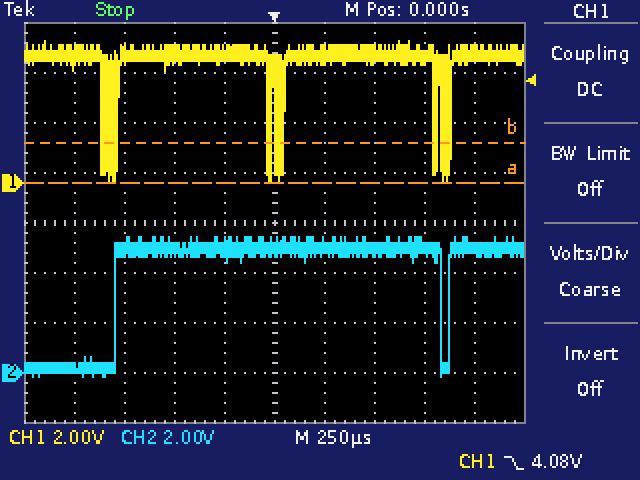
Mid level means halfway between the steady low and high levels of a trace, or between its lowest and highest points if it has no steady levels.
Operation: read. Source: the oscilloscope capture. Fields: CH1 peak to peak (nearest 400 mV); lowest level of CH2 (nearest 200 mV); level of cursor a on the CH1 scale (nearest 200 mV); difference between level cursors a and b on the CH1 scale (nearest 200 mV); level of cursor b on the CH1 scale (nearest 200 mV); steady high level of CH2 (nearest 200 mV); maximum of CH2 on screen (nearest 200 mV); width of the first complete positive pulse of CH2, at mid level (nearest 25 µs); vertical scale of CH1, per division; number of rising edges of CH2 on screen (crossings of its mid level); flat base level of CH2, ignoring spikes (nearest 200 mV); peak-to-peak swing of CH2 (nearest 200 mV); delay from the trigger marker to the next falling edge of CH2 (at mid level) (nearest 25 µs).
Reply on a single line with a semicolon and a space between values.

5.6 V; -200 mV; 0.0 V; 1.6 V; 1.6 V; 5.0 V; 5.4 V; 1.625 ms; 2 V; 2; 200 mV; 5.6 V; 825 µs
